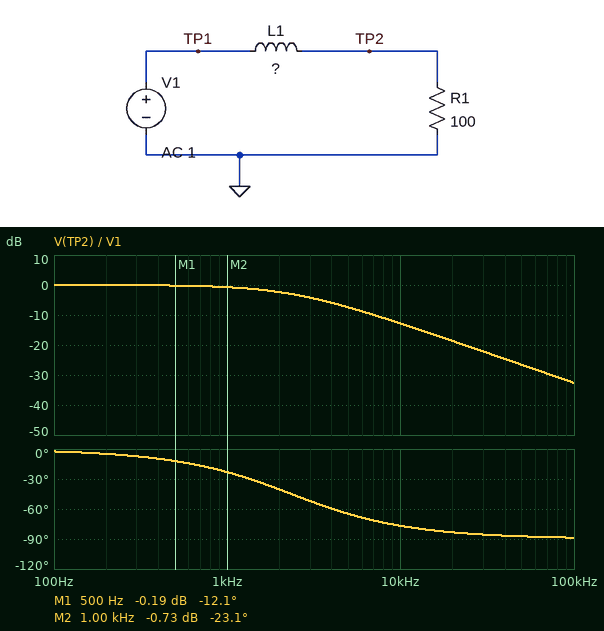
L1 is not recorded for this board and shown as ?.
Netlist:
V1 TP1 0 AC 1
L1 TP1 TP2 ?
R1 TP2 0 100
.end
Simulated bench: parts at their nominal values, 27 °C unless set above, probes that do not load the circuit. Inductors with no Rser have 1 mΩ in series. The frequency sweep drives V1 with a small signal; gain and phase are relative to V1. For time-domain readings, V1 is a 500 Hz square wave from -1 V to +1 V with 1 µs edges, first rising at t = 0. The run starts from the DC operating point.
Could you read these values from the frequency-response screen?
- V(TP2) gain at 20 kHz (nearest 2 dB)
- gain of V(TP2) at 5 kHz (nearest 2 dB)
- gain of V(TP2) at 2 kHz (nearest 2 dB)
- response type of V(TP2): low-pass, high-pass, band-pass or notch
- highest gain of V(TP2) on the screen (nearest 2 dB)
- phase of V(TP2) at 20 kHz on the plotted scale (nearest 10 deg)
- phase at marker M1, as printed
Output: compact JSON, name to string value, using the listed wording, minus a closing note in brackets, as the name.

{"V(TP2) gain at 20 kHz": "-18 dB", "gain of V(TP2) at 5 kHz": "-8 dB", "gain of V(TP2) at 2 kHz": "-2 dB", "response type of V(TP2): low-pass, high-pass, band-pass or notch": "low-pass", "highest gain of V(TP2) on the screen": "0 dB", "phase of V(TP2) at 20 kHz on the plotted scale": "-80 deg", "phase at marker M1, as printed": "-12.1 deg"}
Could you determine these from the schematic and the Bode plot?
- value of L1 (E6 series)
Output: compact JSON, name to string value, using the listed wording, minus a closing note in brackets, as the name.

{"value of L1": "6.8 mH"}
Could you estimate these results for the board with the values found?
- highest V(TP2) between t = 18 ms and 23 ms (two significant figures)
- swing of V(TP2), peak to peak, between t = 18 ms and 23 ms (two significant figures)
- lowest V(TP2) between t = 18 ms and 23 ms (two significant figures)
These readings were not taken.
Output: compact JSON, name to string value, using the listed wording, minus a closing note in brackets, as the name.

{"highest V(TP2) between t = 18 ms and 23 ms": "1.0 V", "swing of V(TP2), peak to peak, between t = 18 ms and 23 ms": "2.0 V", "lowest V(TP2) between t = 18 ms and 23 ms": "-1.0 V"}
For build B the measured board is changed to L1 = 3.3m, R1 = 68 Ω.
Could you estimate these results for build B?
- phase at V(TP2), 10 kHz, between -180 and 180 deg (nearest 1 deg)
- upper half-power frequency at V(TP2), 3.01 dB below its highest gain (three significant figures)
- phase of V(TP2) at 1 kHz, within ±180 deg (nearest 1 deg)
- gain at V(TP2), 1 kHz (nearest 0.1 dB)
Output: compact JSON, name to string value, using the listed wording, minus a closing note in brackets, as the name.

{"phase at V(TP2), 10 kHz, between -180 and 180 deg": "-72 deg", "upper half-power frequency at V(TP2), 3.01 dB below its highest gain": "3.28 kHz", "phase of V(TP2) at 1 kHz, within ±180 deg": "-17 deg", "gain at V(TP2), 1 kHz": "-0.4 dB"}
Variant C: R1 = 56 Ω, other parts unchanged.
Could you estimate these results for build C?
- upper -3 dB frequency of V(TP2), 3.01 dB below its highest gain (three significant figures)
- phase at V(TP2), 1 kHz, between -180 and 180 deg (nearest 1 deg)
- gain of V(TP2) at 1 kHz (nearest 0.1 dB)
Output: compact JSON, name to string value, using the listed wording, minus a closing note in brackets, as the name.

{"upper -3 dB frequency of V(TP2), 3.01 dB below its highest gain": "1.31 kHz", "phase at V(TP2), 1 kHz, between -180 and 180 deg": "-37 deg", "gain of V(TP2) at 1 kHz": "-2.0 dB"}
